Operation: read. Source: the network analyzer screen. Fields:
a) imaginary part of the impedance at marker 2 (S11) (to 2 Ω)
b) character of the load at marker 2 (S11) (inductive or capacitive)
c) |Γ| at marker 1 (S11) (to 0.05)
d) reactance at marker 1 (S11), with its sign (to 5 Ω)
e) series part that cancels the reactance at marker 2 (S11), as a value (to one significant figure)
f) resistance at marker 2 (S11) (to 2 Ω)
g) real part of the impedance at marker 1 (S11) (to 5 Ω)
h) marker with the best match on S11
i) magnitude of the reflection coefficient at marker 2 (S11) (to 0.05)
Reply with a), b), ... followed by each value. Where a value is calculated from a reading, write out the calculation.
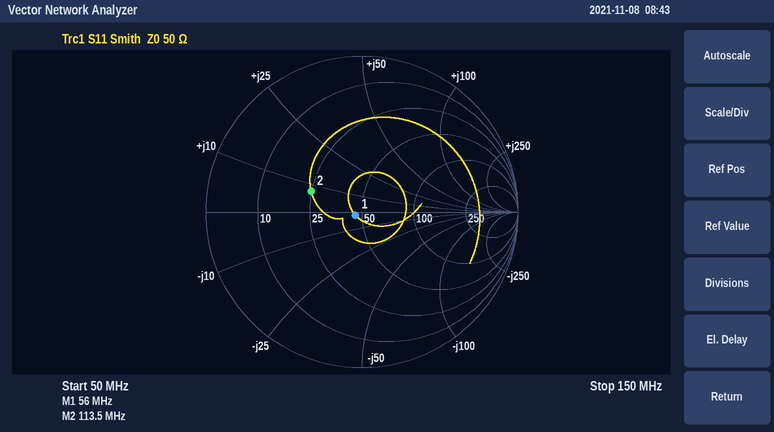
a) +8 Ω
b) inductive
c) 0.05
d) 0 Ω
e) C = 1/(2π × 113.5 MHz × 8 Ω) ≈ 175 pF, so 200 pF to one significant figure
f) 24 Ω
g) 45 Ω
h) marker 1
i) 0.35
